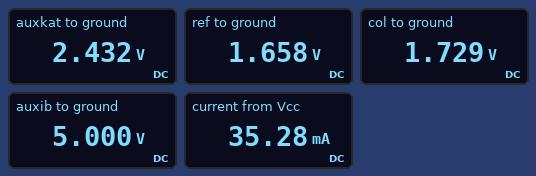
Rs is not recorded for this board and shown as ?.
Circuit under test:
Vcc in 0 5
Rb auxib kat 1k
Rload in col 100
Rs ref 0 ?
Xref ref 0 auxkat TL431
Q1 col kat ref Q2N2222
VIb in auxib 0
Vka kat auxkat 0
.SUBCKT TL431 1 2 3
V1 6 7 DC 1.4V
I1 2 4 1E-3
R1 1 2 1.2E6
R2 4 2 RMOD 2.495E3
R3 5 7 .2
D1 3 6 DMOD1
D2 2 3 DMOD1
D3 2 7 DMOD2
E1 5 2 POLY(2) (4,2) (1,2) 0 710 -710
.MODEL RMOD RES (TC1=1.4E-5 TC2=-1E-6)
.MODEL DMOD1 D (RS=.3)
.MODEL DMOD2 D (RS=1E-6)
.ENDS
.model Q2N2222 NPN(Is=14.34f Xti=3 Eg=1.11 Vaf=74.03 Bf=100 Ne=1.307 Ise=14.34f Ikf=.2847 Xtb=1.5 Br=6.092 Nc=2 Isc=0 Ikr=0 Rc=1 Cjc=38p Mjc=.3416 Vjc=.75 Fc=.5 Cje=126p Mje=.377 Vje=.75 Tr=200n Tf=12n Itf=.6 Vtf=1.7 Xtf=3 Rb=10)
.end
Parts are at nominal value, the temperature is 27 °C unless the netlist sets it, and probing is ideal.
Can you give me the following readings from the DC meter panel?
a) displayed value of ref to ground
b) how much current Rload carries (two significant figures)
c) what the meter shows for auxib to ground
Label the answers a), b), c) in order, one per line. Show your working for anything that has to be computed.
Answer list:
a) 1.658 V
b) (5 V - 1.729 V) / 100 Ω = 33 mA
c) 5.000 V
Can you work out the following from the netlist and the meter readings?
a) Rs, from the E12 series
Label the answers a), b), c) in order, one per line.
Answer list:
a) 47 Ω
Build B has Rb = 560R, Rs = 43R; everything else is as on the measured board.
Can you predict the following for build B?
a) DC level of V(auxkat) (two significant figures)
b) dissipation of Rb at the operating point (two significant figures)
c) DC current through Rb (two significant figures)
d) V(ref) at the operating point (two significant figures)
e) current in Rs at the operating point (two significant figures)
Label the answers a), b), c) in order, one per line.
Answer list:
a) 2.4 V
b) 12 mW
c) 4.6 mA
d) 1.6 V
e) 38 mA
